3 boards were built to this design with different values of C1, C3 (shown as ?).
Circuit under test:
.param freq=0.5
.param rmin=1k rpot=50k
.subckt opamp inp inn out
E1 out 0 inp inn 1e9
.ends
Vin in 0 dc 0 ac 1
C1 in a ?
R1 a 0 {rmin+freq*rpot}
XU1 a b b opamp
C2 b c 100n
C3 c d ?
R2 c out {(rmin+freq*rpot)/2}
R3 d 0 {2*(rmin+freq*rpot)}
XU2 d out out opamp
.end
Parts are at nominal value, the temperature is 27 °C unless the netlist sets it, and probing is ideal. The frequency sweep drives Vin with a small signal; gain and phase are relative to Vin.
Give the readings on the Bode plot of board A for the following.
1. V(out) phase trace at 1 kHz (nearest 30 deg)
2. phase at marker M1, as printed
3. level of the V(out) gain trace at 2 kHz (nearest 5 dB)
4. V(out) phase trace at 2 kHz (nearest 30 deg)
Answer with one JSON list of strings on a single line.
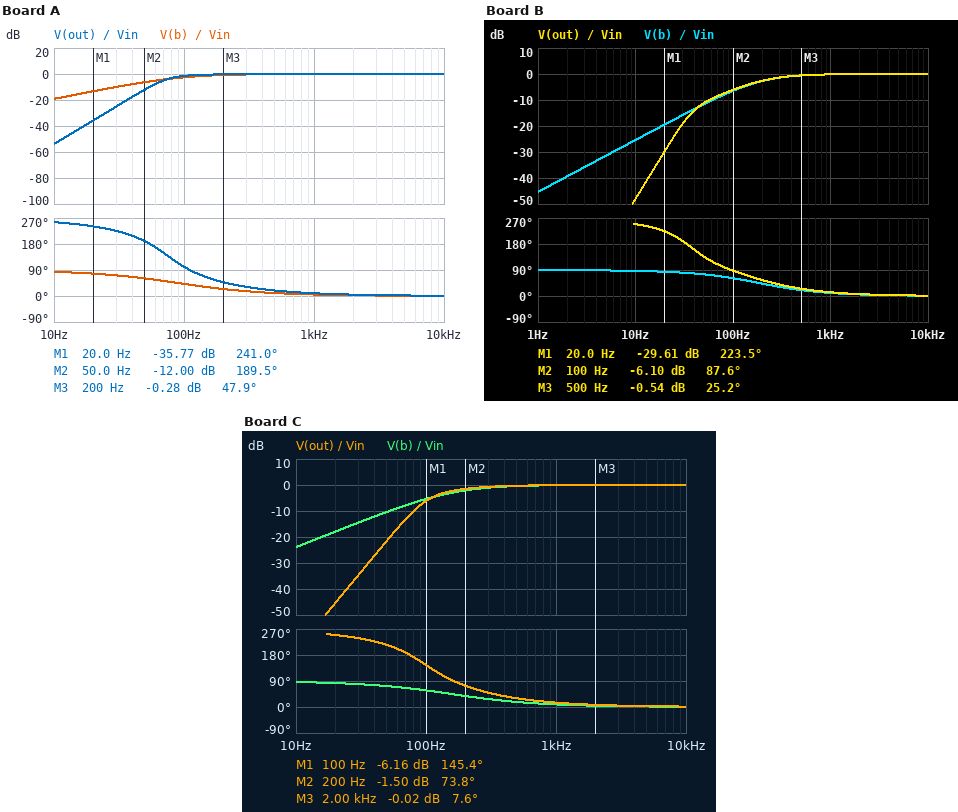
["0 deg", "241.0 deg", "0 dB", "0 deg"]
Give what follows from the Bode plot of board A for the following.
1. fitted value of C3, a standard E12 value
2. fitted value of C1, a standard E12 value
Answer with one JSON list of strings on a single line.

["68 nF", "68 nF"]
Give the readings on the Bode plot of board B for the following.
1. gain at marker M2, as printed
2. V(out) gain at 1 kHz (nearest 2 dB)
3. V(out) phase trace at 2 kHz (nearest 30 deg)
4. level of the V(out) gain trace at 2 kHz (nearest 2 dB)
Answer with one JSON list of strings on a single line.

["-6.10 dB", "0 dB", "0 deg", "0 dB"]
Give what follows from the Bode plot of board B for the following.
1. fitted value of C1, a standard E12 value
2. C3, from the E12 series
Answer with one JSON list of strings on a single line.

["33 nF", "270 nF"]
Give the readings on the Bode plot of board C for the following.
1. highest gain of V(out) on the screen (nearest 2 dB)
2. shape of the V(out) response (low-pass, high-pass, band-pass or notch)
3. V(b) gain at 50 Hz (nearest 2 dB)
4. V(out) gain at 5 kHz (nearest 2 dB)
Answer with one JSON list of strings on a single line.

["0 dB", "high-pass", "-10 dB", "0 dB"]
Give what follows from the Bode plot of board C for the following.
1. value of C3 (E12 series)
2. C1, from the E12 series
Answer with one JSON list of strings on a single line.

["39 nF", "39 nF"]
